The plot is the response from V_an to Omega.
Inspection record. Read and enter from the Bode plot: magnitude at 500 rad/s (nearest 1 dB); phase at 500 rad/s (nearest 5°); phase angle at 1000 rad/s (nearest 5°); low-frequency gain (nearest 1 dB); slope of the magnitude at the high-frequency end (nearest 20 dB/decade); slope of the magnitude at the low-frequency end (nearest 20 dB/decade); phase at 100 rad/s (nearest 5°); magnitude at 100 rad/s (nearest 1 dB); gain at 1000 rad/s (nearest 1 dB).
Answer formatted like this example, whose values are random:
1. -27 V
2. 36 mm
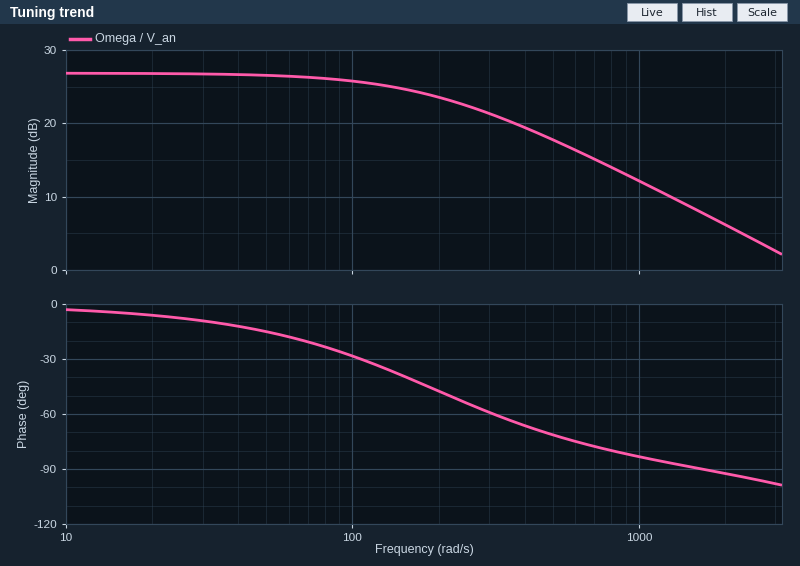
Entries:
1. 18 dB
2. -70°
3. -85°
4. 27 dB
5. -20 dB/decade
6. 0 dB/decade
7. -30°
8. 26 dB
9. 12 dB
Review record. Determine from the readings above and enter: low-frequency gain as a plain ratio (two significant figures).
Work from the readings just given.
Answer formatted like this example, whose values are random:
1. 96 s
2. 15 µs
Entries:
1. 22
